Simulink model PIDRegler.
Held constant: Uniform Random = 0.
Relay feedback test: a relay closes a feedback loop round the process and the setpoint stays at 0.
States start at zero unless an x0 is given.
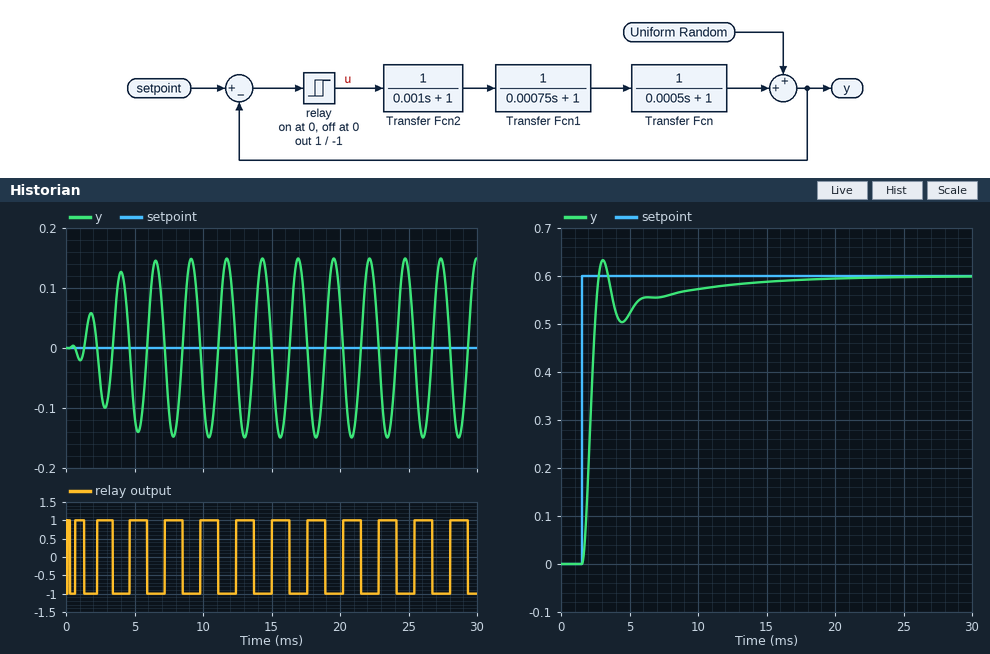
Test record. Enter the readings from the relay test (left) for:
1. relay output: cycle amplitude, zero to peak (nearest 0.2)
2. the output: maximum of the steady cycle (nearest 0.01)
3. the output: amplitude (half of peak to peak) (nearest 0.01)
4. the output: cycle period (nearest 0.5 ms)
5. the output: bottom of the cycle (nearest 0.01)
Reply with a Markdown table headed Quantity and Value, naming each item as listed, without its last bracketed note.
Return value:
| Quantity | Value |
|---|---|
| relay output: cycle amplitude, zero to peak | 1.0 |
| the output: maximum of the steady cycle | 0.15 |
| the output: amplitude (half of peak to peak) | 0.15 |
| the output: cycle period | 2.5 ms |
| the output: bottom of the cycle | -0.15 |
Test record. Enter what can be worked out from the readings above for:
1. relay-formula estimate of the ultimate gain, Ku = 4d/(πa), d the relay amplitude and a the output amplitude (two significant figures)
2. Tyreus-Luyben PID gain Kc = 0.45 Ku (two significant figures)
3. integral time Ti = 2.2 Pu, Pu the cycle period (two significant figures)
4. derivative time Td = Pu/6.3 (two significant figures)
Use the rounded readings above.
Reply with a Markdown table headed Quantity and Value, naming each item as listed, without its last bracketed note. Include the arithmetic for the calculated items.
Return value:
| Quantity | Value |
|---|---|
| relay-formula estimate of the ultimate gain, Ku = 4d/(πa), d the relay amplitude and a the output amplitude | 4 × 1 / (π × 0.15) = 8.5 |
| Tyreus-Luyben PID gain Kc = 0.45 Ku | 0.45 × 8.5 = 3.8 |
| integral time Ti = 2.2 Pu, Pu the cycle period | 2.2 × 2.5 = 5.5 ms |
| derivative time Td = Pu/6.3 | 2.5 / 6.3 = 0.40 ms |
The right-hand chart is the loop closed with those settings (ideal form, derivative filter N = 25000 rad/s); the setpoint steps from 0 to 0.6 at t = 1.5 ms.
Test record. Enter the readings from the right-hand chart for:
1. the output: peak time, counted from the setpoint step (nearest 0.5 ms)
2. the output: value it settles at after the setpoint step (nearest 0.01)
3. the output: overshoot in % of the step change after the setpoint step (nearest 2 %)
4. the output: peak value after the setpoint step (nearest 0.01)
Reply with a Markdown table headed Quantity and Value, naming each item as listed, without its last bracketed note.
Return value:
| Quantity | Value |
|---|---|
| the output: peak time, counted from the setpoint step | 1.5 ms |
| the output: value it settles at after the setpoint step | 0.60 |
| the output: overshoot in % of the step change after the setpoint step | 6 % |
| the output: peak value after the setpoint step | 0.63 |
